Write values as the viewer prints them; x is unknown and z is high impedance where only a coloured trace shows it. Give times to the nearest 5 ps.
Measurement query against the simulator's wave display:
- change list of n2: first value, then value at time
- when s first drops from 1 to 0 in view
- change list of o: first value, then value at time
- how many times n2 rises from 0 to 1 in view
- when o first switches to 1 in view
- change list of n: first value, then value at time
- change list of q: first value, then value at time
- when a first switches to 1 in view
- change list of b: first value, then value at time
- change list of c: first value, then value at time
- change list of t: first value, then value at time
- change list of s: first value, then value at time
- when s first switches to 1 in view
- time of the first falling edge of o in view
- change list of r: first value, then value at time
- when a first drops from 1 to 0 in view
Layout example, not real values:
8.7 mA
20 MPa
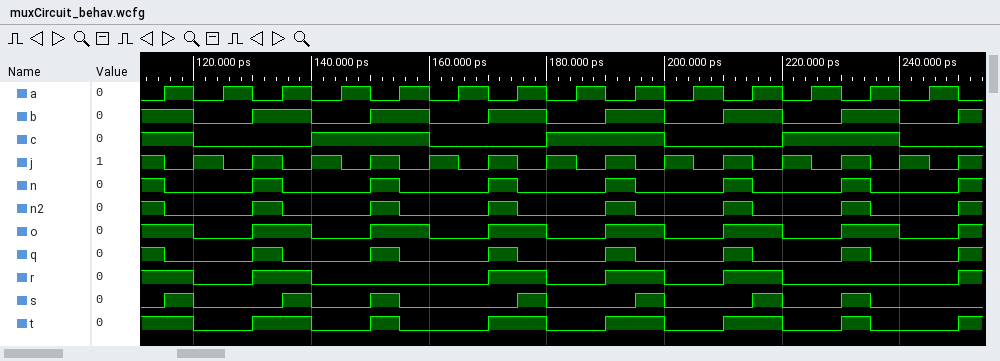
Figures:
1, 0 at 115 ps, 1 at 130 ps, 0 at 135 ps, 1 at 150 ps, 0 at 155 ps, 1 at 170 ps, 0 at 175 ps, 1 at 190 ps, 0 at 195 ps, 1 at 210 ps, 0 at 215 ps, 1 at 230 ps, 0 at 235 ps, 1 at 250 ps
120 ps
1, 0 at 120 ps, 1 at 130 ps, 0 at 140 ps, 1 at 150 ps, 0 at 160 ps, 1 at 170 ps, 0 at 180 ps, 1 at 190 ps, 0 at 200 ps, 1 at 210 ps, 0 at 220 ps, 1 at 230 ps, 0 at 240 ps, 1 at 250 ps
7
130 ps
1, 0 at 115 ps, 1 at 130 ps, 0 at 135 ps, 1 at 150 ps, 0 at 155 ps, 1 at 170 ps, 0 at 175 ps, 1 at 190 ps, 0 at 195 ps, 1 at 210 ps, 0 at 215 ps, 1 at 230 ps, 0 at 235 ps, 1 at 250 ps
1, 0 at 115 ps, 1 at 130 ps, 0 at 135 ps, 1 at 150 ps, 0 at 155 ps, 1 at 170 ps, 0 at 175 ps, 1 at 190 ps, 0 at 195 ps, 1 at 210 ps, 0 at 215 ps, 1 at 230 ps, 0 at 235 ps, 1 at 250 ps
115 ps
1, 0 at 120 ps, 1 at 130 ps, 0 at 140 ps, 1 at 150 ps, 0 at 160 ps, 1 at 170 ps, 0 at 180 ps, 1 at 190 ps, 0 at 200 ps, 1 at 210 ps, 0 at 220 ps, 1 at 230 ps, 0 at 240 ps, 1 at 250 ps
1, 0 at 120 ps, 1 at 140 ps, 0 at 160 ps, 1 at 180 ps, 0 at 200 ps, 1 at 220 ps, 0 at 240 ps
1, 0 at 120 ps, 1 at 130 ps, 0 at 140 ps, 1 at 150 ps, 0 at 155 ps, 1 at 170 ps, 0 at 180 ps, 1 at 190 ps, 0 at 200 ps, 1 at 210 ps, 0 at 220 ps, 1 at 230 ps, 0 at 235 ps, 1 at 250 ps
0, 1 at 115 ps, 0 at 120 ps, 1 at 135 ps, 0 at 140 ps, 1 at 150 ps, 0 at 155 ps, 1 at 175 ps, 0 at 180 ps, 1 at 195 ps, 0 at 200 ps, 1 at 215 ps, 0 at 220 ps, 1 at 230 ps, 0 at 235 ps
115 ps
120 ps
1, 0 at 120 ps, 1 at 130 ps, 0 at 140 ps, 1 at 170 ps, 0 at 180 ps, 1 at 190 ps, 0 at 200 ps, 1 at 210 ps, 0 at 220 ps, 1 at 250 ps
120 ps
